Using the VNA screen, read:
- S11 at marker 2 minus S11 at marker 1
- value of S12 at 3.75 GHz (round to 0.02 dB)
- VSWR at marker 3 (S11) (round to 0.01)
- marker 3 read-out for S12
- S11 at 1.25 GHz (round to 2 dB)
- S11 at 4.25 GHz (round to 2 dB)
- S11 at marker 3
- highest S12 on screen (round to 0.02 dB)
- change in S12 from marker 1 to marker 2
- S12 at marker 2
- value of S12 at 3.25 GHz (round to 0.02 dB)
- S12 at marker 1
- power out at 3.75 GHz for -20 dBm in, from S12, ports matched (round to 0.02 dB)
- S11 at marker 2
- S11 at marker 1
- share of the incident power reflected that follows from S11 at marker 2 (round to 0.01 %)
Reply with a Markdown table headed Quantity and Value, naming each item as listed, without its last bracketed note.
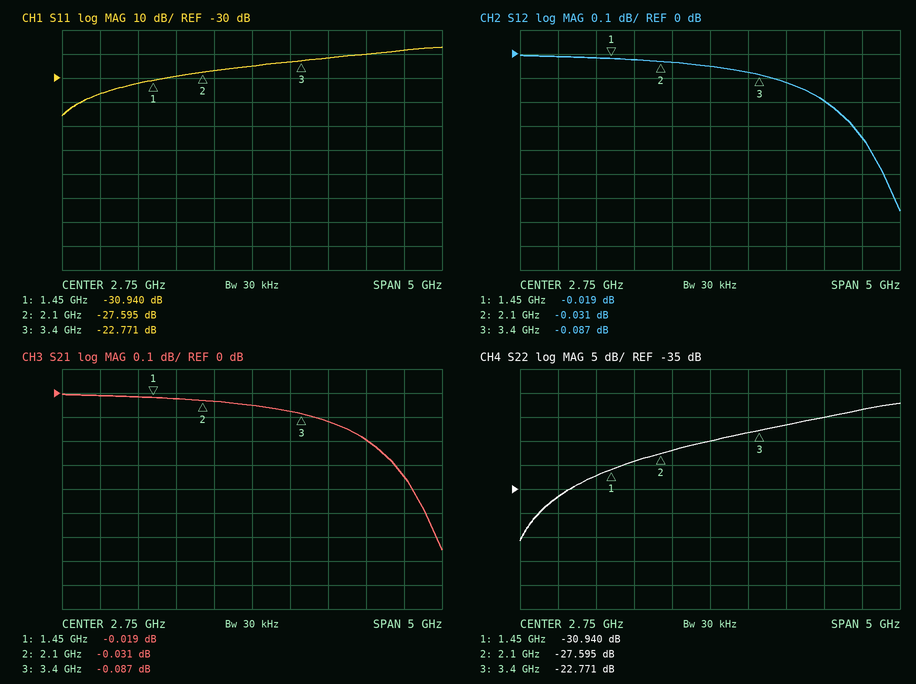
| Quantity | Value |
|---|---|
| S11 at marker 2 minus S11 at marker 1 | 3.345 dB |
| value of S12 at 3.75 GHz | -0.12 dB |
| VSWR at marker 3 (S11) | 1.16 |
| marker 3 read-out for S12 | -0.087 dB |
| S11 at 1.25 GHz | -32 dB |
| S11 at 4.25 GHz | -20 dB |
| S11 at marker 3 | -22.771 dB |
| highest S12 on screen | 0.00 dB |
| change in S12 from marker 1 to marker 2 | -0.012 dB |
| S12 at marker 2 | -0.031 dB |
| value of S12 at 3.25 GHz | -0.08 dB |
| S12 at marker 1 | -0.019 dB |
| power out at 3.75 GHz for -20 dBm in, from S12, ports matched | -20.12 dBm |
| S11 at marker 2 | -27.595 dB |
| S11 at marker 1 | -30.940 dB |
| share of the incident power reflected that follows from S11 at marker 2 | 0.17 % |
